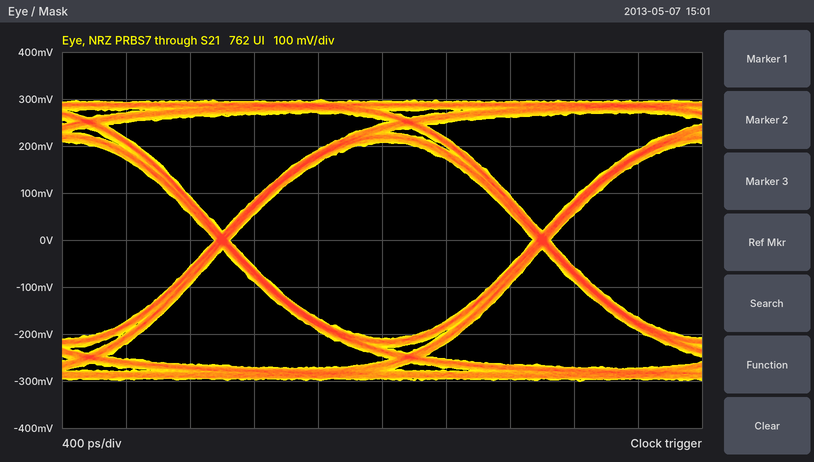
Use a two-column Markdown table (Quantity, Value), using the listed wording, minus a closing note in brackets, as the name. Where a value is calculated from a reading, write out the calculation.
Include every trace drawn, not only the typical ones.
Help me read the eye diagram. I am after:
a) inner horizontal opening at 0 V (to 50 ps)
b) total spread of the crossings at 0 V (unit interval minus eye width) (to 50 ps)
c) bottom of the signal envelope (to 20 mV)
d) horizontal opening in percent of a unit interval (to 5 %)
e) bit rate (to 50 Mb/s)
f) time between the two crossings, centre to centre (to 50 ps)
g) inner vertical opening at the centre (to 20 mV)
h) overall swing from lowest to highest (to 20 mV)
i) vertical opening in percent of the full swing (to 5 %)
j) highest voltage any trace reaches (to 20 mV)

| Quantity | Value |
|---|---|
| inner horizontal opening at 0 V | 1.90 ns |
| total spread of the crossings at 0 V (unit interval minus eye width) | 100 ps |
| bottom of the signal envelope | -300 mV |
| horizontal opening in percent of a unit interval | 1.90 ns / 2.00 ns ≈ 95 % |
| bit rate | 500 Mb/s |
| time between the two crossings, centre to centre | 2.00 ns |
| inner vertical opening at the centre | 420 mV |
| overall swing from lowest to highest | 600 mV |
| vertical opening in percent of the full swing | 420 mV / 600 mV ≈ 70 % |
| highest voltage any trace reaches | 300 mV |
